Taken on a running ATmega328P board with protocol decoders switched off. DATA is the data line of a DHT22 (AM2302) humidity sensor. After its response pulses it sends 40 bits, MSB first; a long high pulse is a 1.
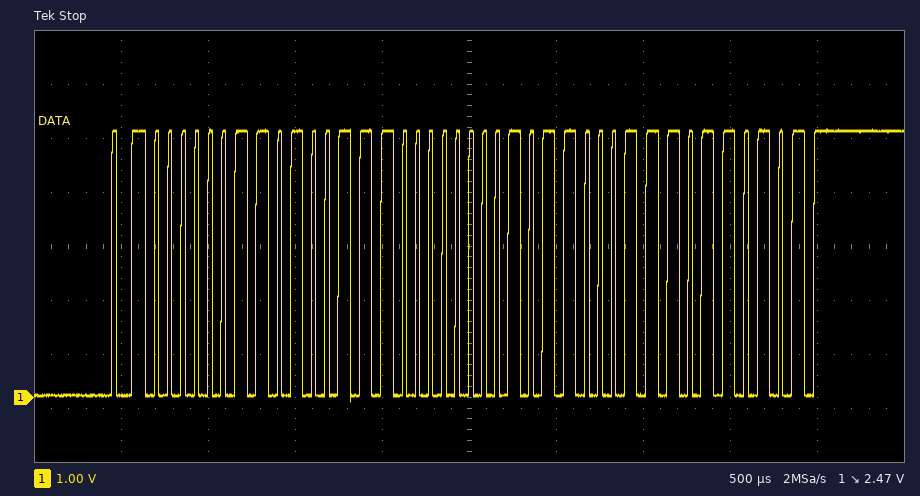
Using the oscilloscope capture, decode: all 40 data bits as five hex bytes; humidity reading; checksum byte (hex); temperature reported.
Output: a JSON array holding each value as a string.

["03 4E 01 63 B5", "84.6 %", "0xB5", "35.5 °C"]
